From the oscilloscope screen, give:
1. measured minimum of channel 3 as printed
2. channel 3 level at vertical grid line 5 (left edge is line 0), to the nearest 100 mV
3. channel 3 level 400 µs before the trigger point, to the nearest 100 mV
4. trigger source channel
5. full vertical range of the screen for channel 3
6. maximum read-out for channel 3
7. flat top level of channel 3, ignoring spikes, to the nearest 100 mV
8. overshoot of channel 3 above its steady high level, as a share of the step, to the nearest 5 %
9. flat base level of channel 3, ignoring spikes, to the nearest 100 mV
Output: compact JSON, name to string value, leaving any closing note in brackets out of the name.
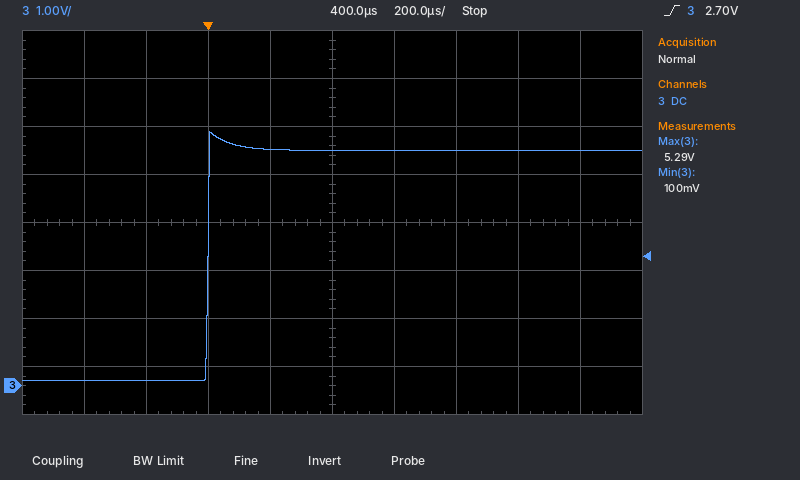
{"measured minimum of channel 3 as printed": "100 mV", "channel 3 level at vertical grid line 5 (left edge is line 0), to the nearest 100 mV": "4.9 V", "channel 3 level 400 µs before the trigger point, to the nearest 100 mV": "100 mV", "trigger source channel": "channel 3", "full vertical range of the screen for channel 3": "8 V", "maximum read-out for channel 3": "5.29 V", "flat top level of channel 3, ignoring spikes, to the nearest 100 mV": "4.9 V", "overshoot of channel 3 above its steady high level, as a share of the step, to the nearest 5 %": "10 %", "flat base level of channel 3, ignoring spikes, to the nearest 100 mV": "100 mV"}
